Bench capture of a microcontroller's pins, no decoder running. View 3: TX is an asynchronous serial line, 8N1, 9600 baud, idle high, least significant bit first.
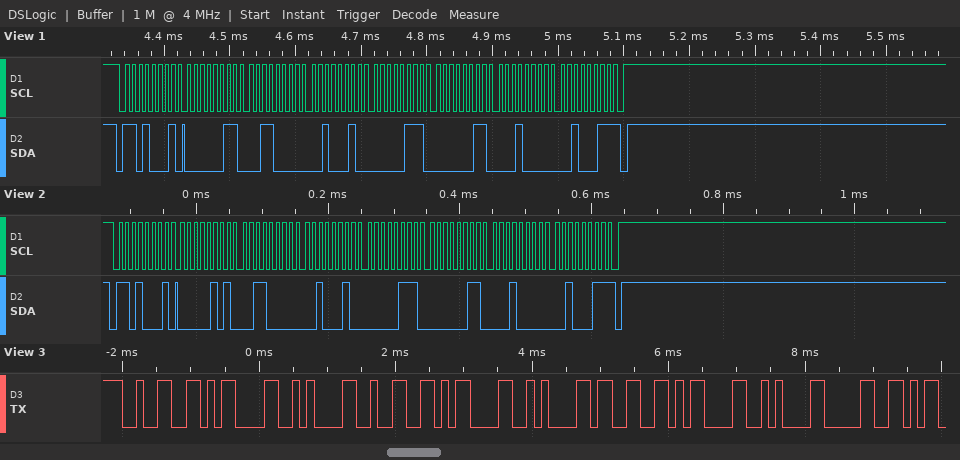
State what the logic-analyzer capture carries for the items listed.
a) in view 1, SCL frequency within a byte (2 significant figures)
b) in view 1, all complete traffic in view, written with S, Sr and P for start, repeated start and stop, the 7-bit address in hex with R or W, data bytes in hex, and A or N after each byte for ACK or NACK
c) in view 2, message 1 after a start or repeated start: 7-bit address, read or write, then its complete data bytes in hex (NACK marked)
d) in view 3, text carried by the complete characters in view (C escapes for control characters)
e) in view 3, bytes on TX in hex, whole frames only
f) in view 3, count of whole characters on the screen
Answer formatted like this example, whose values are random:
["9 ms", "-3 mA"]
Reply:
["100 kHz", "S 68R A 03 A 30 A 22 A 07 A 03 A 10 A 23 N P", "0x68 read: 05 30 22 07 03 10 23 NACK", "\"2\\r\\n2\\r\\n3\\r\\n0\"", "32 0D 0A 32 0D 0A 33 0D 0A 30", "10"]
